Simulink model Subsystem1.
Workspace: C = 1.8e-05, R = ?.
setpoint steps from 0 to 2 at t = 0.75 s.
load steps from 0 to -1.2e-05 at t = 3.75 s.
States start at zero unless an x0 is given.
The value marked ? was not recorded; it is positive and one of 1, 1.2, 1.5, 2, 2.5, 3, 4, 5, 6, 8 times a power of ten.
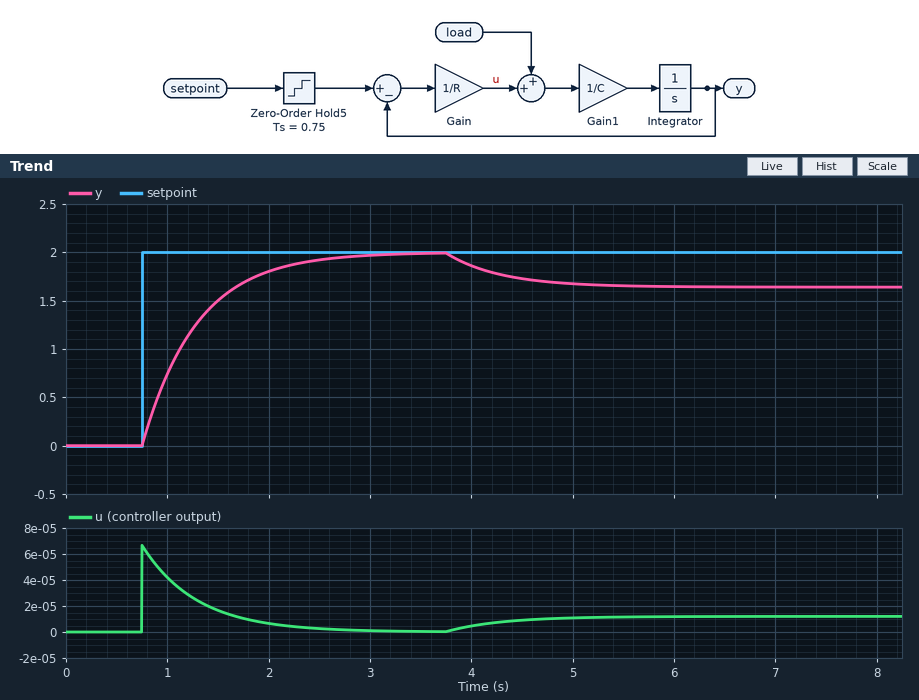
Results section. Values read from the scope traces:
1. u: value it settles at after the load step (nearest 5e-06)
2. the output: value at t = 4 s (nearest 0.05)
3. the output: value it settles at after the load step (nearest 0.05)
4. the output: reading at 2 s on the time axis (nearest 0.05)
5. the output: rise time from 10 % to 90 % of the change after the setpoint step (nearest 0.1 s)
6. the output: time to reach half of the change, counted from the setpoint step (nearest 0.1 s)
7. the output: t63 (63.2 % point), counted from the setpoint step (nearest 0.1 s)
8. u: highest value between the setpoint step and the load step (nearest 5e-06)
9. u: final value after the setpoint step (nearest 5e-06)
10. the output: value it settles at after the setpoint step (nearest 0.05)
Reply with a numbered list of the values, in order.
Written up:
1. 0.000010
2. 1.85
3. 1.65
4. 1.80
5. 1.2 s
6. 0.4 s
7. 0.5 s
8. 0.000065
9. 0.000000
10. 2.00
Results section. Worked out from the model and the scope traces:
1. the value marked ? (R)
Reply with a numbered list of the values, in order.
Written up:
1. 30000
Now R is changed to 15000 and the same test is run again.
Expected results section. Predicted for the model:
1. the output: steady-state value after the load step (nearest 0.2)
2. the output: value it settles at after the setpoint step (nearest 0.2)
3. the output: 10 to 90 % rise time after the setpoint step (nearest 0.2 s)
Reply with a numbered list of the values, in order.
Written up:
1. 1.8
2. 2.0
3. 0.6 s
